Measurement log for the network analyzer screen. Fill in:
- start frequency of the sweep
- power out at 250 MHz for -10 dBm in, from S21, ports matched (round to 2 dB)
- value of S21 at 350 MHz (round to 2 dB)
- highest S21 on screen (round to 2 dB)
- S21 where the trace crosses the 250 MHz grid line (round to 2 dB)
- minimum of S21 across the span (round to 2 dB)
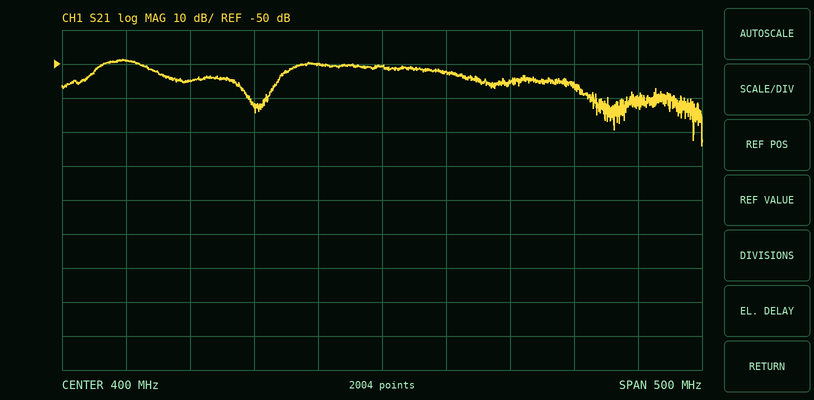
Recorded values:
150 MHz
-64 dBm
-50 dB
-48 dB
-54 dB
-74 dB
